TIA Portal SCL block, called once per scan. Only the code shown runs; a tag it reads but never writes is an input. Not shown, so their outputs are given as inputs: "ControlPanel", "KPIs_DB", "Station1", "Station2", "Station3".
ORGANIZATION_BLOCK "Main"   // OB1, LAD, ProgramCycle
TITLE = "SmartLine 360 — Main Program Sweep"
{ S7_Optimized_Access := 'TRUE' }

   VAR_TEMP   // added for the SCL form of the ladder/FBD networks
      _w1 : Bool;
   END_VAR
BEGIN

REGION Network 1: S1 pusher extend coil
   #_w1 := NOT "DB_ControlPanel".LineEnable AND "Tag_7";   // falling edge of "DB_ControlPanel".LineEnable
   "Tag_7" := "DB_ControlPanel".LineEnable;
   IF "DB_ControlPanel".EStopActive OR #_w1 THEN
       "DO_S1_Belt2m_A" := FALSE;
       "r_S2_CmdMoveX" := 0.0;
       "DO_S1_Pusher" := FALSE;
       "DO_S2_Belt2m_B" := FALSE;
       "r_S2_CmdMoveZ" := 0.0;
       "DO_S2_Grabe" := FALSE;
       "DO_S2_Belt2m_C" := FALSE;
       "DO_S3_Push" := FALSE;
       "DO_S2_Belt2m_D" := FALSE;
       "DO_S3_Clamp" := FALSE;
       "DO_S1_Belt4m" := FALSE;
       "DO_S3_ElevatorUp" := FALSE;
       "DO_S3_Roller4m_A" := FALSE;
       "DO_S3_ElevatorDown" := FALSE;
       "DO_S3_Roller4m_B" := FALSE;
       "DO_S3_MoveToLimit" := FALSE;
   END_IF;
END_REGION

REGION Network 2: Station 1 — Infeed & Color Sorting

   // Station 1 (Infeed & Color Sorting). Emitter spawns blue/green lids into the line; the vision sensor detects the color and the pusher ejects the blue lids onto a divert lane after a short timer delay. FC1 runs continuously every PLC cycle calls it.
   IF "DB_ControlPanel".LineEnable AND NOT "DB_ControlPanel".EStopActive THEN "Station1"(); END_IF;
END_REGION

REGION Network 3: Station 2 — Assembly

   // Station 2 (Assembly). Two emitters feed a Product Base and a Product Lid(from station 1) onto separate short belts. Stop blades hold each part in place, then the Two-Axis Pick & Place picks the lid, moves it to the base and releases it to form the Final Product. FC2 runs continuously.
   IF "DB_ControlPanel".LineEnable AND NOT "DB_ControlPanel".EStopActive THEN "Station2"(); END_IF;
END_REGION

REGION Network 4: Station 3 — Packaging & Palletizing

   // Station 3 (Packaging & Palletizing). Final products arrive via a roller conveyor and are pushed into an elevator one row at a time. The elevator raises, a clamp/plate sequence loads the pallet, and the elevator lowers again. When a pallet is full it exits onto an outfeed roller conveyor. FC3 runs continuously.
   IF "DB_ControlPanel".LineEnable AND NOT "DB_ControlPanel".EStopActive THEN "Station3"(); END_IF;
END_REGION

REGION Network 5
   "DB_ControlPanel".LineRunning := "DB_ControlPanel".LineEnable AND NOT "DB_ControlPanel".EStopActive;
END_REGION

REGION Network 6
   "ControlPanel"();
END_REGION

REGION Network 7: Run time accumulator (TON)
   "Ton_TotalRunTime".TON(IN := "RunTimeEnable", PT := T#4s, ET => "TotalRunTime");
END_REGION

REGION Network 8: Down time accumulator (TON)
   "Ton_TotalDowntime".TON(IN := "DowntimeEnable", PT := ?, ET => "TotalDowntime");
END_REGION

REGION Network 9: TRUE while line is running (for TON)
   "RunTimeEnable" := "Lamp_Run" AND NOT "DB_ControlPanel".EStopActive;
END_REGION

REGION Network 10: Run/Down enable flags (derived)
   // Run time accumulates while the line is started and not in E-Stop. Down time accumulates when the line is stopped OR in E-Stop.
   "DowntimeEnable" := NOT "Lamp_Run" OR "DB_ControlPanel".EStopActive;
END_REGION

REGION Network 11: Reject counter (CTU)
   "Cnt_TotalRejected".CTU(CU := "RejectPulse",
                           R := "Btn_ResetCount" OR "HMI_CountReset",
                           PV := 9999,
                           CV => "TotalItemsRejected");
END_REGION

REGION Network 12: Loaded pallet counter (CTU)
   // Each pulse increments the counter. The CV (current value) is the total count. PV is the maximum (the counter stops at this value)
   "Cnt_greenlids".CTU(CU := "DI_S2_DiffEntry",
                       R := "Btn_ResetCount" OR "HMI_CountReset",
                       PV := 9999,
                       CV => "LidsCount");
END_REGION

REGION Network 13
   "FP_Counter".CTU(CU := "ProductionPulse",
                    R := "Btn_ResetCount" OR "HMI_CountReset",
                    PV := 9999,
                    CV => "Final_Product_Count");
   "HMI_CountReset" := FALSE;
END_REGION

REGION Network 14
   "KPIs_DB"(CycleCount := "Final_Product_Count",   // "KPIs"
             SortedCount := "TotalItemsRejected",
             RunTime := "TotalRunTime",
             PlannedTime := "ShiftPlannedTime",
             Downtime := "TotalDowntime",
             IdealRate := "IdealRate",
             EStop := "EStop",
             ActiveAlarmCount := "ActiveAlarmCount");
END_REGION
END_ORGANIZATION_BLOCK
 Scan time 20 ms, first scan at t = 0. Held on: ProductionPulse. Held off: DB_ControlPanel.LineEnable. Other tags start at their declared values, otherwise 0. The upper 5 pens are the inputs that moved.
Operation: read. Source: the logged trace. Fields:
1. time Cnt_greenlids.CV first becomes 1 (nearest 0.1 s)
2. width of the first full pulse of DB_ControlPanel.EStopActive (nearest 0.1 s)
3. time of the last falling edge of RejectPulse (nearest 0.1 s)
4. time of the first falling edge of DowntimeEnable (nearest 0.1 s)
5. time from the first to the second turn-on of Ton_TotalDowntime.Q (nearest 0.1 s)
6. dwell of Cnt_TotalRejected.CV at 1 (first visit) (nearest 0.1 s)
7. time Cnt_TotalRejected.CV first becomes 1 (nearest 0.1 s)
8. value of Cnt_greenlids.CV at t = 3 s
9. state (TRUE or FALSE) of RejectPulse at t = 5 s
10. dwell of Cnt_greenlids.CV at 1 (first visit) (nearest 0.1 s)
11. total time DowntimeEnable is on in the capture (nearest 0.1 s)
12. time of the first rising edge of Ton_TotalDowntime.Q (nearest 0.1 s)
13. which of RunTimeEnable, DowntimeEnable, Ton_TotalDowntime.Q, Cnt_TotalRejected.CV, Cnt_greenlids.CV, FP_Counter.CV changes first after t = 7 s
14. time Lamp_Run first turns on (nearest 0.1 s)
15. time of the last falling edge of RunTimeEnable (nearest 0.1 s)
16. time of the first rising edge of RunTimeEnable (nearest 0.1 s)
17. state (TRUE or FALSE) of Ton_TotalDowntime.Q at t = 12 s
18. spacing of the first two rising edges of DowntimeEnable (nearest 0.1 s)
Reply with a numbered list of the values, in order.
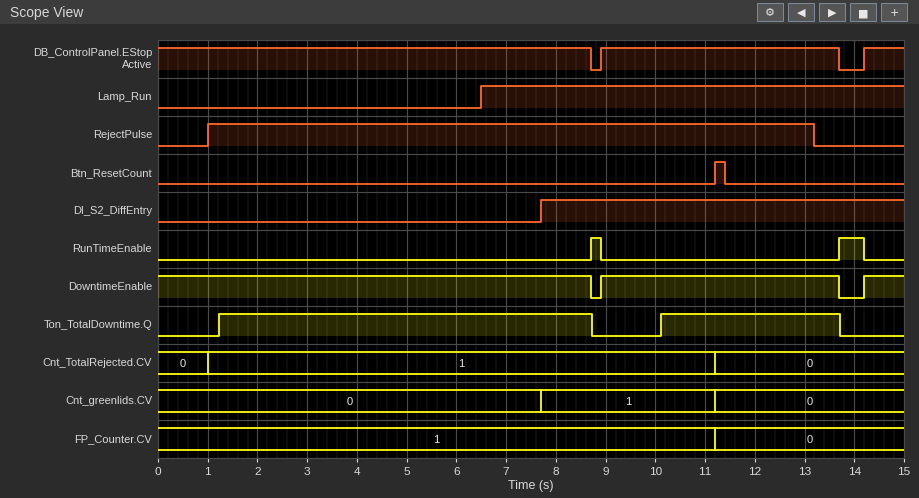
1. 7.7 s
2. 4.8 s
3. 13.2 s
4. 8.7 s
5. 8.9 s
6. 10.2 s
7. 1.0 s
8. 0
9. TRUE
10. 3.5 s
11. 14.3 s
12. 1.2 s
13. Cnt_greenlids.CV
14. 6.5 s
15. 14.2 s
16. 8.7 s
17. TRUE
18. 5.3 s
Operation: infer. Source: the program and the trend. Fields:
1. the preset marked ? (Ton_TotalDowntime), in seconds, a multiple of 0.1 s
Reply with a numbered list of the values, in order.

1. 1.2 s
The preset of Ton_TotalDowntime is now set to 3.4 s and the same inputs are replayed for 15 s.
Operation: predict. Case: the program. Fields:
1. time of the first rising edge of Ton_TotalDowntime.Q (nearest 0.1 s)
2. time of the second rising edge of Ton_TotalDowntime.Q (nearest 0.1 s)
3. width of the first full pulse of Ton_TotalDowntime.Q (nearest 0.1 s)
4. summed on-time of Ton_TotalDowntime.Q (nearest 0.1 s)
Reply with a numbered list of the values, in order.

1. 3.4 s
2. 12.3 s
3. 5.3 s
4. 6.7 s
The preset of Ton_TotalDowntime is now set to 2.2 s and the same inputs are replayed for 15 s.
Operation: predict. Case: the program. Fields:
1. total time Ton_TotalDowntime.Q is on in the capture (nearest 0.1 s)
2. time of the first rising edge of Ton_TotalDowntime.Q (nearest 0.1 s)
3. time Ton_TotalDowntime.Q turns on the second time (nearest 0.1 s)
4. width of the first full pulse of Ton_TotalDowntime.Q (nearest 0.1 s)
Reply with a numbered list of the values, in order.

1. 9.1 s
2. 2.2 s
3. 11.1 s
4. 6.5 s
